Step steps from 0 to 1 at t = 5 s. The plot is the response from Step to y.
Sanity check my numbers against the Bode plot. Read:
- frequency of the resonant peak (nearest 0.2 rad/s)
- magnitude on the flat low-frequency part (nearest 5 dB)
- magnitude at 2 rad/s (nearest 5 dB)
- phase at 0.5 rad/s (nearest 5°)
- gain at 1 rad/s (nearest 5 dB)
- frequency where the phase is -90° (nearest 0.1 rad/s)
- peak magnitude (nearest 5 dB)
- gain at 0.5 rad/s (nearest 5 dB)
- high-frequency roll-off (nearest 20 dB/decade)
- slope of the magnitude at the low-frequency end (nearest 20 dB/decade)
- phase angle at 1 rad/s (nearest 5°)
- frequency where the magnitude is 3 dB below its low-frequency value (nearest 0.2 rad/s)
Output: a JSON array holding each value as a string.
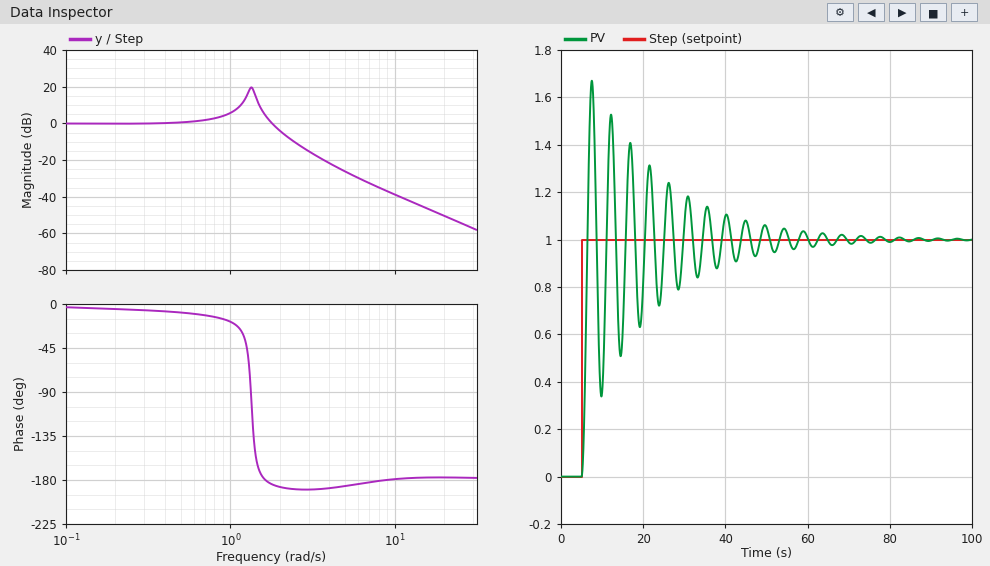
["1.4 rad/s", "0 dB", "-5 dB", "-10°", "5 dB", "1.3 rad/s", "20 dB", "0 dB", "-40 dB/decade", "0 dB/decade", "-20°", "2.0 rad/s"]
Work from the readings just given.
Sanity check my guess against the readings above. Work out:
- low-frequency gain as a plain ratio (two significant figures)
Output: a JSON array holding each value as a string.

["1.0"]
